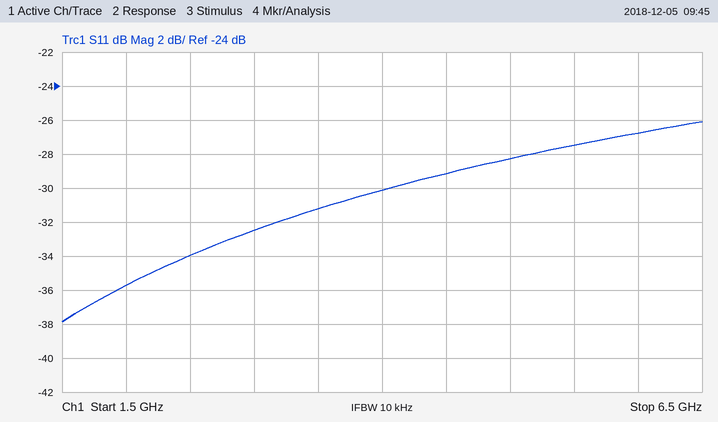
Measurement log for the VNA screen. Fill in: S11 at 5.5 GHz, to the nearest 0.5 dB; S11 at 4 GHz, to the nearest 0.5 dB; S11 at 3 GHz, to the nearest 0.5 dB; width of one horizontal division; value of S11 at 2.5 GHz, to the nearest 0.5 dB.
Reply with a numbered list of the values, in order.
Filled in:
1. -27.5 dB
2. -30.0 dB
3. -32.5 dB
4. 500 MHz
5. -34.0 dB
